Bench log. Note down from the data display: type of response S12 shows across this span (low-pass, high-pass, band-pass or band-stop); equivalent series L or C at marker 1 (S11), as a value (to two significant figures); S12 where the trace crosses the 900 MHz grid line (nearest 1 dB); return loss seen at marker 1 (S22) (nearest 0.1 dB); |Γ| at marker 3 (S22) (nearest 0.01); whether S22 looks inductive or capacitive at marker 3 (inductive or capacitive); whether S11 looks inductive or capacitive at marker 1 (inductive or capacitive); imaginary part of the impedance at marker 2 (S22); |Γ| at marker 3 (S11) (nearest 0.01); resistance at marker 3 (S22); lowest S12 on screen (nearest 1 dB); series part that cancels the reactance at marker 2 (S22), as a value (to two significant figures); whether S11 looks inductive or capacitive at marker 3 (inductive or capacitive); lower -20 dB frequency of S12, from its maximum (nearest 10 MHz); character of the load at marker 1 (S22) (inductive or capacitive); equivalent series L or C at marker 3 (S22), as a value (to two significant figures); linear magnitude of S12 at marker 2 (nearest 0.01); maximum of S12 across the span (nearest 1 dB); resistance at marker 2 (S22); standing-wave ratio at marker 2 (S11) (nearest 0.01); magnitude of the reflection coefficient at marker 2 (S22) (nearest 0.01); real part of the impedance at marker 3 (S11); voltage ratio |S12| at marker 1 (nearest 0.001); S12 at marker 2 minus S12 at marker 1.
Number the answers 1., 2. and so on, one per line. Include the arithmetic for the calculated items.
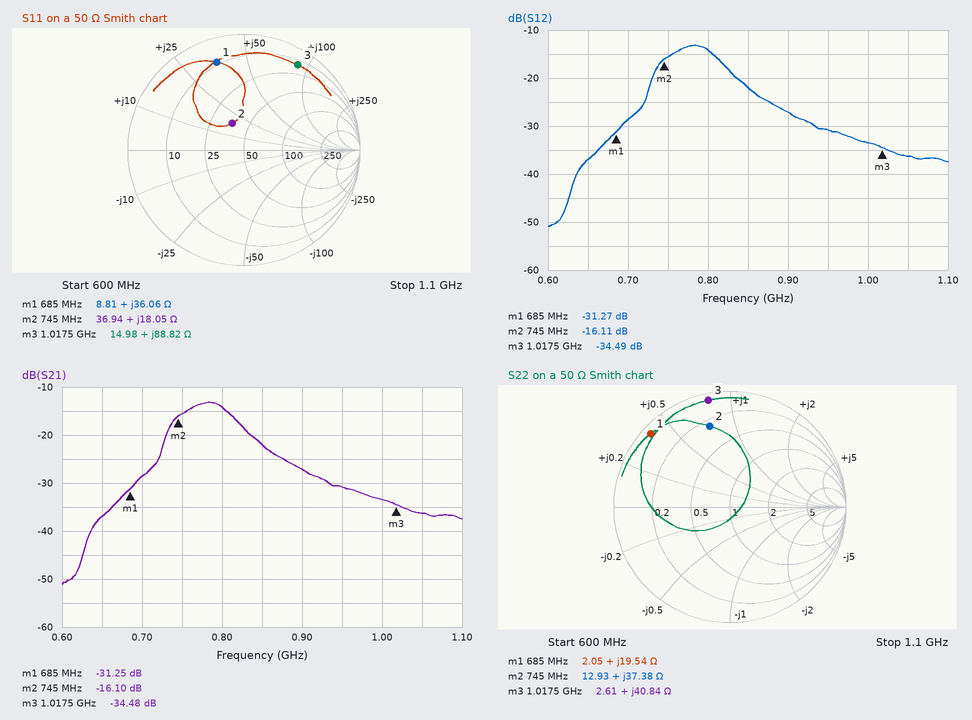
1. band-pass
2. L = 36.06 Ω/(2π × 685 MHz) ≈ 8.4 nH
3. -27 dB
4. 0.6 dB
5. 0.94
6. inductive
7. inductive
8. +37.38 Ω
9. 0.87
10. 2.61 Ω
11. -51 dB
12. C = 1/(2π × 745 MHz × 37.38 Ω) ≈ 5.7 pF
13. inductive
14. 670 MHz
15. inductive
16. L = 40.84 Ω/(2π × 1.0175 GHz) ≈ 6.4 nH
17. 10^(-16.11/20) ≈ 0.16
18. -13 dB
19. 12.93 Ω
20. 1.67
21. 0.72
22. 14.98 Ω
23. 10^(-31.27/20) ≈ 0.027
24. -16.11 − (-31.27) = 15.16 dB
